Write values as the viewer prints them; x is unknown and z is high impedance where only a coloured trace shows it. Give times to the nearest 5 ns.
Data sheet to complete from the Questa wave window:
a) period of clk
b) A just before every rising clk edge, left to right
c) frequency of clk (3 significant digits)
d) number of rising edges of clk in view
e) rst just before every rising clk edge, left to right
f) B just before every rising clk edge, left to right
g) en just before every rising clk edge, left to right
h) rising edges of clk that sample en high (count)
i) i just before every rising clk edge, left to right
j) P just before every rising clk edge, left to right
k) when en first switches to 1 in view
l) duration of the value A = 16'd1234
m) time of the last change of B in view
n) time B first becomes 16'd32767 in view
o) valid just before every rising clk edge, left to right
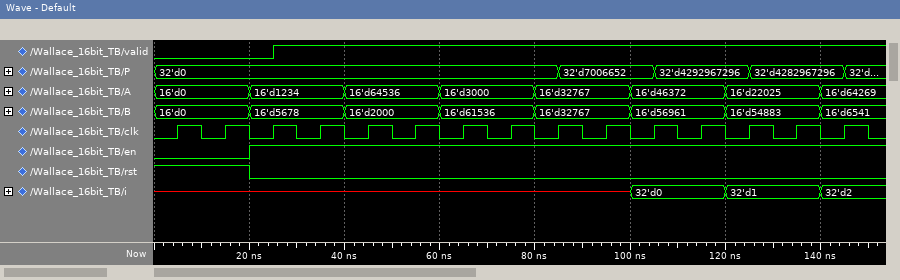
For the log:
10 ns
16'd0, 16'd0, 16'd1234, 16'd1234, 16'd64536, 16'd64536, 16'd3000, 16'd3000, 16'd32767, 16'd32767, 16'd46372, 16'd46372, 16'd22025, 16'd22025, 16'd64269
100 MHz
15
1 1 0 0 0 0 0 0 0 0 0 0 0 0 0
16'd0, 16'd0, 16'd5678, 16'd5678, 16'd2000, 16'd2000, 16'd61536, 16'd61536, 16'd32767, 16'd32767, 16'd56961, 16'd56961, 16'd54883, 16'd54883, 16'd6541
0 0 1 1 1 1 1 1 1 1 1 1 1 1 1
13
x, x, x, x, x, x, x, x, x, x, 32'd0, 32'd0, 32'd1, 32'd1, 32'd2
32'd0, 32'd0, 32'd0, 32'd0, 32'd0, 32'd0, 32'd0, 32'd0, 32'd0, 32'd7006652, 32'd7006652, 32'd4292967296, 32'd4292967296, 32'd4282967296, 32'd4282967296
20 ns
20 ns
140 ns
80 ns
0 0 0 1 1 1 1 1 1 1 1 1 1 1 1
